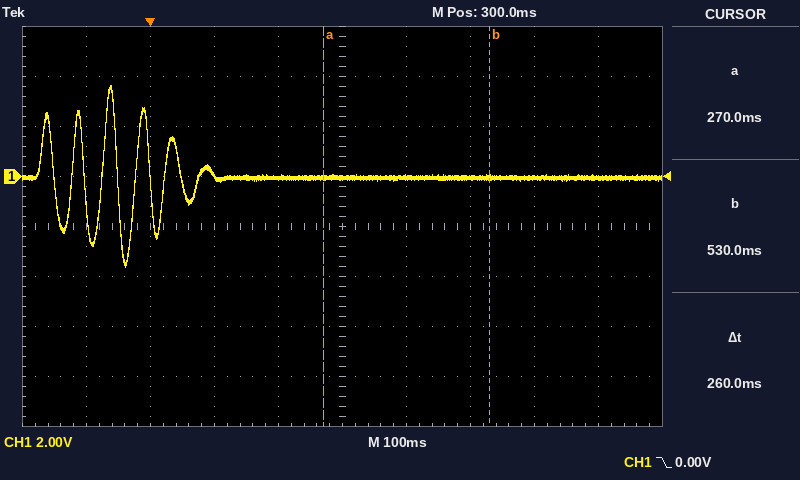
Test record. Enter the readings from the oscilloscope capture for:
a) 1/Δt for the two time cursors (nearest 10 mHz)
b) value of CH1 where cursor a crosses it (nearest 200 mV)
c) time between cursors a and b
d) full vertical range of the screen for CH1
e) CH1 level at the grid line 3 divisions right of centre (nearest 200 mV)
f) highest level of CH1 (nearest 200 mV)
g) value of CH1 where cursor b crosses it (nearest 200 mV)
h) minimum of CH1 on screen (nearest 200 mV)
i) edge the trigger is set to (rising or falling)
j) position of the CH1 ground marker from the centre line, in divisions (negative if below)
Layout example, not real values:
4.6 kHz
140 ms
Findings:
3.85 Hz
0.0 V
260 ms
16 V
0.0 V
3.6 V
0.0 V
-3.6 V
falling
+1.0 div
